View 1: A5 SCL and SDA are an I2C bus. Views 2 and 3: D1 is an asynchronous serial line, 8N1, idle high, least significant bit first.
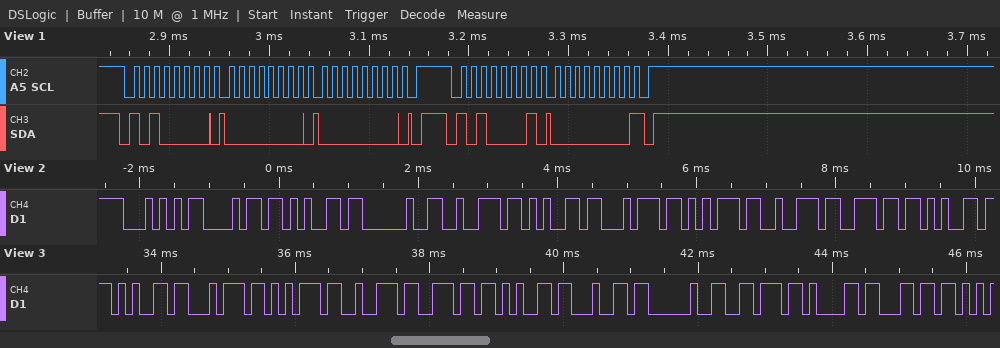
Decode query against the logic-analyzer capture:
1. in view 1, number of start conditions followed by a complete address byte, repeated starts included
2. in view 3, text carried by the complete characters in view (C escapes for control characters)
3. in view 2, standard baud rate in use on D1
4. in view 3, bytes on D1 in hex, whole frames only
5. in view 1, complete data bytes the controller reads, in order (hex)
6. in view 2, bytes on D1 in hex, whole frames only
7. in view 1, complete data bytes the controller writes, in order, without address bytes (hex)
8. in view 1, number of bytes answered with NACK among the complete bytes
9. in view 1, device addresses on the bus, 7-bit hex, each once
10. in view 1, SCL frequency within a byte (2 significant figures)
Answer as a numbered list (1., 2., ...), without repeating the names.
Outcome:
1. 2
2. "eturned val"
3. 9600 baud
4. 0x65 0x74 0x75 0x72 0x6E 0x65 0x64 0x20 0x76 0x61 0x6C
5. 00
6. 54 68 65 20 72 65 74 75 72 6E 65
7. 00 00
8. 1
9. 0x50
10. 100 kHz
